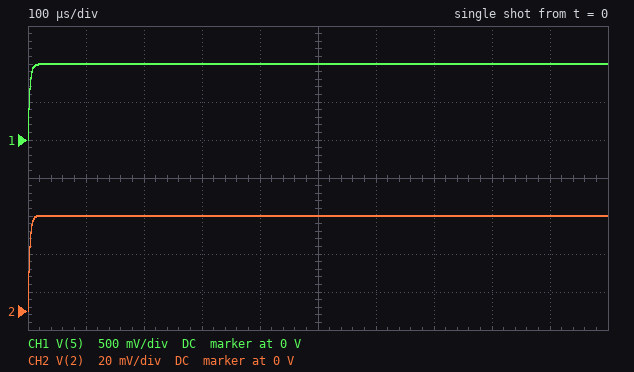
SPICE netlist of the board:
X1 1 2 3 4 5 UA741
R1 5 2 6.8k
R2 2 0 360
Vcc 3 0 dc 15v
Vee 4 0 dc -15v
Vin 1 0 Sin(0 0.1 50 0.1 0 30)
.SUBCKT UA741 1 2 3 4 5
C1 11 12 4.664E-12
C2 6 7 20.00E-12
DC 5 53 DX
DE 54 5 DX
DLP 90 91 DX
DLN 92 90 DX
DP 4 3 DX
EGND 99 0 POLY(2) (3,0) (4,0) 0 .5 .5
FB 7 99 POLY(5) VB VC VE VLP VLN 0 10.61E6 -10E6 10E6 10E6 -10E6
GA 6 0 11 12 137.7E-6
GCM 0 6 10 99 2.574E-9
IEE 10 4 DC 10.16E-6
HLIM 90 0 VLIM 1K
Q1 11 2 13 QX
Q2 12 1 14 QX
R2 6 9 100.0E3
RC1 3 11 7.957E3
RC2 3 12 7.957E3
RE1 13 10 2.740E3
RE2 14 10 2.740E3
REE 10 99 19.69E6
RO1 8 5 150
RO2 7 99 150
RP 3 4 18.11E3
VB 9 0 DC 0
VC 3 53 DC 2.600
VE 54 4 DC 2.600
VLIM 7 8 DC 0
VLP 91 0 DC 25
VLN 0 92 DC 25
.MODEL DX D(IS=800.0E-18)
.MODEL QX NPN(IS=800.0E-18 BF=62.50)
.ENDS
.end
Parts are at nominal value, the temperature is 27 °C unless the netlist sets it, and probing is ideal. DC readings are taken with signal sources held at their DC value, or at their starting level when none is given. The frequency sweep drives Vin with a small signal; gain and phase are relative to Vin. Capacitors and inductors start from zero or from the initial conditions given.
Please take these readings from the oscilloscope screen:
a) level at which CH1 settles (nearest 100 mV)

1.0 V
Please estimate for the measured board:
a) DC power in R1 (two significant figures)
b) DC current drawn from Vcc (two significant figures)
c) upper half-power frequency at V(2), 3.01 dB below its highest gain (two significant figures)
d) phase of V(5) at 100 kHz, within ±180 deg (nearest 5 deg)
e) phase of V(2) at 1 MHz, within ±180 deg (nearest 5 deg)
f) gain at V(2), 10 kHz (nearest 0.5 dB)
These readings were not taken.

130 µW
1.7 mA
55 kHz
-65 deg
-110 deg
0 dB
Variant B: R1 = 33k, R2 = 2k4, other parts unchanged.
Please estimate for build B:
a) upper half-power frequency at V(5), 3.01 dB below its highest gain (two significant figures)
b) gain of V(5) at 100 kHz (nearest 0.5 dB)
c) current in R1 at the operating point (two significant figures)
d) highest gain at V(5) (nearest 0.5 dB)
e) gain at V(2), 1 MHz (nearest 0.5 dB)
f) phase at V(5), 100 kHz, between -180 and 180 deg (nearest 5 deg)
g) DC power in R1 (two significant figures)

76 kHz
19.0 dB
21 µA
23.5 dB
-23.5 dB
-55 deg
14 µW
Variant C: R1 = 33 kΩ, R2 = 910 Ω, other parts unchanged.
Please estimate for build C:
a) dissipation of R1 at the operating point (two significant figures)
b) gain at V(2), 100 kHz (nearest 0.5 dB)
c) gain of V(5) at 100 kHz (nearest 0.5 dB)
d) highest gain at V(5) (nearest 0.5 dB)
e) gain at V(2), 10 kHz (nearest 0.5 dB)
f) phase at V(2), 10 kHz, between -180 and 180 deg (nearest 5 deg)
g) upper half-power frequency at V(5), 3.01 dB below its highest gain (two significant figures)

100 µW
-11.0 dB
20.5 dB
31.5 dB
-0.5 dB
-20 deg
30 kHz
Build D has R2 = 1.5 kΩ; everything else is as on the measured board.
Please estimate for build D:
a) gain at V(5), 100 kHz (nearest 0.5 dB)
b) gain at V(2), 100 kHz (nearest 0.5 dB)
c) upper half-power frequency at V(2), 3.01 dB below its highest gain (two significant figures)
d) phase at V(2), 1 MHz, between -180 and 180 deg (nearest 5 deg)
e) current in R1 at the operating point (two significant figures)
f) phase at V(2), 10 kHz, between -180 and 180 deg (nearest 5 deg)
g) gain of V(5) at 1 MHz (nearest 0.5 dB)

14.0 dB
-1.0 dB
210 kHz
-105 deg
33 µA
-5 deg
0.5 dB
